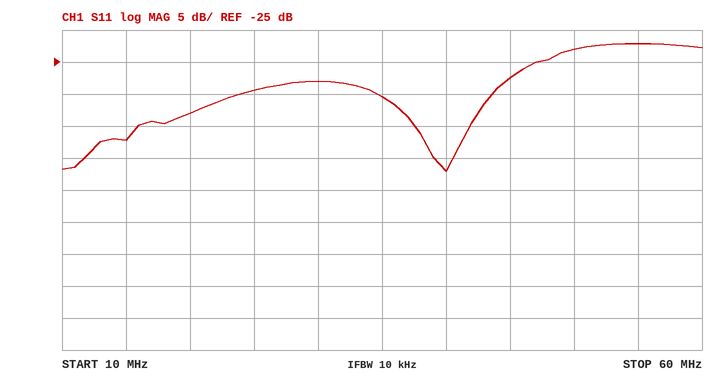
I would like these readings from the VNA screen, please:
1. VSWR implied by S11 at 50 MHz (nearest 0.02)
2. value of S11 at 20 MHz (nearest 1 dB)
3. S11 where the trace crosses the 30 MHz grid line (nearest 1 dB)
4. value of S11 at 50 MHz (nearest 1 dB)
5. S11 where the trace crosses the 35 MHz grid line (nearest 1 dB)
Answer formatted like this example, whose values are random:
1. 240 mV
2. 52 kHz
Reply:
1. 1.16
2. -33 dB
3. -28 dB
4. -23 dB
5. -30 dB
